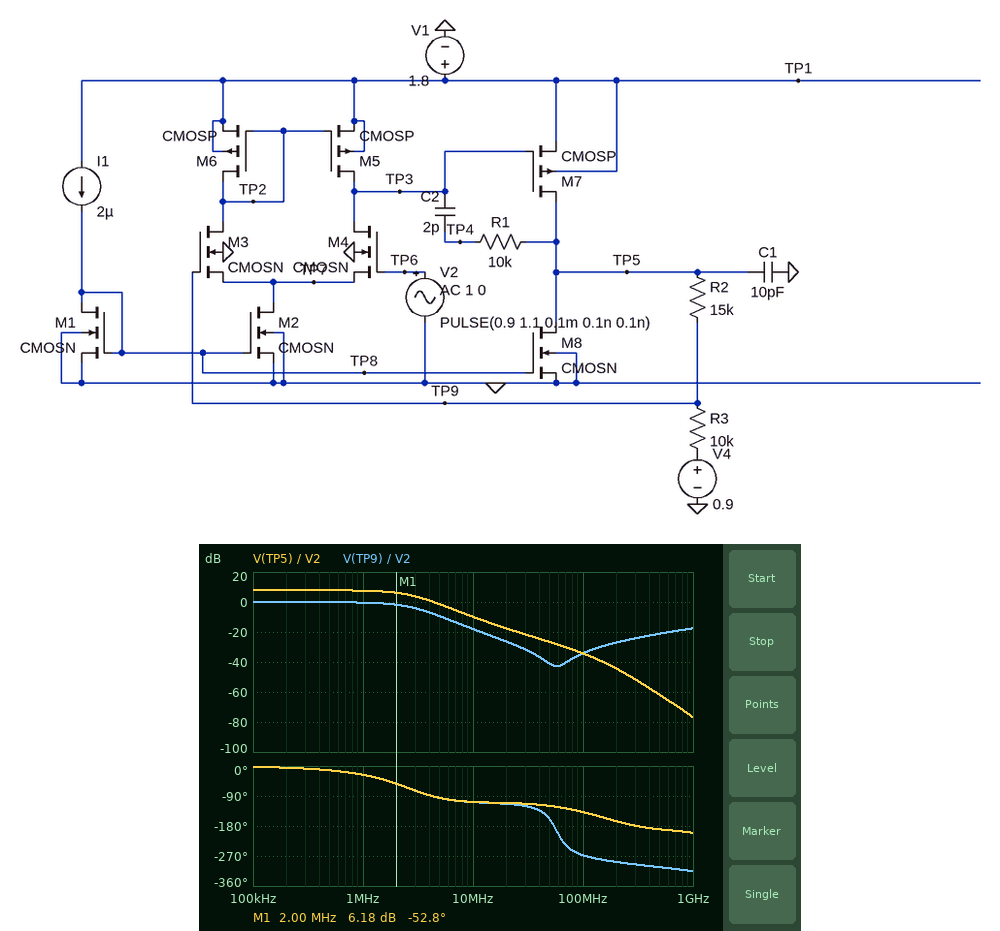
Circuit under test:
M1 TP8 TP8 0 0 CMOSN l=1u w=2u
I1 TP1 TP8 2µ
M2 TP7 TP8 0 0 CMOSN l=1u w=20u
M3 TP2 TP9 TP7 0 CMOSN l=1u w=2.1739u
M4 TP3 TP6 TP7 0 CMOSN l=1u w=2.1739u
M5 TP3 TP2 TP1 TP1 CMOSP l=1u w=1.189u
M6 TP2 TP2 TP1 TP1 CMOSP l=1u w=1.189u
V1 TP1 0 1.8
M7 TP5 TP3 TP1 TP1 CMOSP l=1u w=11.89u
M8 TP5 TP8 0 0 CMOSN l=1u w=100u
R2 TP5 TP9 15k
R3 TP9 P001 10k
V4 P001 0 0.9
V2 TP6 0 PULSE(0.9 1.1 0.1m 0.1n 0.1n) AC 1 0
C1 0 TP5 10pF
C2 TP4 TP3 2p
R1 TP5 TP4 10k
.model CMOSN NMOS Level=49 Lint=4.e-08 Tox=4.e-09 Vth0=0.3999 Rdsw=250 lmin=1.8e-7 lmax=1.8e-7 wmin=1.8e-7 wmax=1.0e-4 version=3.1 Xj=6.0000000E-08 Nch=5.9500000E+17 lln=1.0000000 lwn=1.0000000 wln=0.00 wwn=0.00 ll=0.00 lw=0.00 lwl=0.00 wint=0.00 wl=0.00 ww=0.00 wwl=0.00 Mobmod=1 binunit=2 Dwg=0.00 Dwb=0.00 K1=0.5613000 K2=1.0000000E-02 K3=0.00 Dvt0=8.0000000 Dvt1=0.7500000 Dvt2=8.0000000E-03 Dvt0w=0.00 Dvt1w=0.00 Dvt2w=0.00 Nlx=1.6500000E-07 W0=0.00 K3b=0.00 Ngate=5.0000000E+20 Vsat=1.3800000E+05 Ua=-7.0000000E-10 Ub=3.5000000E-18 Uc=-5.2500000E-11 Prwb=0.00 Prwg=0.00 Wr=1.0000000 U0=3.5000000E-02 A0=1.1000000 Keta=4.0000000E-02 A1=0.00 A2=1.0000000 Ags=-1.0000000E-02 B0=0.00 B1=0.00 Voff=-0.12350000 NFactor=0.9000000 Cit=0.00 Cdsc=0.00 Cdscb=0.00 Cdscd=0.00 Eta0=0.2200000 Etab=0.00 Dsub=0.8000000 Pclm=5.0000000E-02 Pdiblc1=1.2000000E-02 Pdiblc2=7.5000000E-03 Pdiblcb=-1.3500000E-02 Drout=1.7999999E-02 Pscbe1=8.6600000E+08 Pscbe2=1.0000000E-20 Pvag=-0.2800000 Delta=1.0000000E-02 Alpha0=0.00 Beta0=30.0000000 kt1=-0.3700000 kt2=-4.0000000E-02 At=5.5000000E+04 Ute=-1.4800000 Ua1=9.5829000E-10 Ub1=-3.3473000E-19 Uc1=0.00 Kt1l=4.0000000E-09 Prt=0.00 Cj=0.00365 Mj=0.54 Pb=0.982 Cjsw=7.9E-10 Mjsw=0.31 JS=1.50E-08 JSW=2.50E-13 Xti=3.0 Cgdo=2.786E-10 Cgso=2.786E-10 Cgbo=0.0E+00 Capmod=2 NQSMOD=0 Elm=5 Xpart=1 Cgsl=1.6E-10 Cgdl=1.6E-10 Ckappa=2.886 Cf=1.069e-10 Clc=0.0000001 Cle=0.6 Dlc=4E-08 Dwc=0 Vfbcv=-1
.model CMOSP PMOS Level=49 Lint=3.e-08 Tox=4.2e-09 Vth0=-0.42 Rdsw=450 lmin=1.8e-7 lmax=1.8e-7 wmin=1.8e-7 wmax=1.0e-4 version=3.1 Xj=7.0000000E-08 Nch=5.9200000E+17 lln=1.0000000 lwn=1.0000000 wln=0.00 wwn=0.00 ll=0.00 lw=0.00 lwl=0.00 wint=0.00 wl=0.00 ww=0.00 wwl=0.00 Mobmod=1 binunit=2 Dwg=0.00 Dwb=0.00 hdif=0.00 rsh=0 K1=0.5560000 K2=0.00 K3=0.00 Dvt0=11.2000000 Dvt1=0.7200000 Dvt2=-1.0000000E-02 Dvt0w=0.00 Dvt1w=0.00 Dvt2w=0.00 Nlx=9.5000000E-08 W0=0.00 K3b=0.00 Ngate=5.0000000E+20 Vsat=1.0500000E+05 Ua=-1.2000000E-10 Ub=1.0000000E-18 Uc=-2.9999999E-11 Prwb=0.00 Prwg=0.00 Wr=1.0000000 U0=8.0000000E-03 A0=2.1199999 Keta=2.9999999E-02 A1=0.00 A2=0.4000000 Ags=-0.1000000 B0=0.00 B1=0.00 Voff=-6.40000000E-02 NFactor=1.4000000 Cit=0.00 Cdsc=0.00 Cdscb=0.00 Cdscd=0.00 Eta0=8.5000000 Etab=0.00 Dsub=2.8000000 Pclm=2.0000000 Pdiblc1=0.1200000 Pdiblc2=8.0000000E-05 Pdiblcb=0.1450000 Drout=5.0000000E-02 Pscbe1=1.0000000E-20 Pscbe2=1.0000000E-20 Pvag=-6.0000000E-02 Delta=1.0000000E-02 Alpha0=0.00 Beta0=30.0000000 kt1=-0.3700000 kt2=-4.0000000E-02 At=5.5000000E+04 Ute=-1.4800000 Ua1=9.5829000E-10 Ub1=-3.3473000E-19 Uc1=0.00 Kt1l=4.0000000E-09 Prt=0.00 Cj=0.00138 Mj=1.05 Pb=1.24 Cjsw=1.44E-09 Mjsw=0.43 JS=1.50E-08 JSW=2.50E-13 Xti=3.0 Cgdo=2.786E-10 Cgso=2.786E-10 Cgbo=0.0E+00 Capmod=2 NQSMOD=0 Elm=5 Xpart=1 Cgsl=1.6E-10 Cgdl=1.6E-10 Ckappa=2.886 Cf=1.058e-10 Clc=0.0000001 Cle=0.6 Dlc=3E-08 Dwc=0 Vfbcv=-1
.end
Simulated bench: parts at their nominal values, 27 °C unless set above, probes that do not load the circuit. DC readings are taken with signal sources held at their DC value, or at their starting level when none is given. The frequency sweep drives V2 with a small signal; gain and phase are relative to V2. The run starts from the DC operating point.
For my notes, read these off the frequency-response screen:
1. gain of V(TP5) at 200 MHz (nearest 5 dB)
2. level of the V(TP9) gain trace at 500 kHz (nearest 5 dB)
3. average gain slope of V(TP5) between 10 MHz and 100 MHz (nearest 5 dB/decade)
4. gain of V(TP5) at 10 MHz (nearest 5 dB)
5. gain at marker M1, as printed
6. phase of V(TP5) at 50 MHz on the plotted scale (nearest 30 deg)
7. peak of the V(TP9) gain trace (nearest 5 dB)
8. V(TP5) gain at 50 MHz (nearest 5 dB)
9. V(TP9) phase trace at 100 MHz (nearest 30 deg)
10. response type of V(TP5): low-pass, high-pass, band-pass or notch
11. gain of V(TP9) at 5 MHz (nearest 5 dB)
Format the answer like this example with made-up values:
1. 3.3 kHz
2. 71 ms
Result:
1. -45 dB
2. 0 dB
3. -25 dB/decade
4. -10 dB
5. 6.18 dB
6. -120 deg
7. 0 dB
8. -25 dB
9. -270 deg
10. low-pass
11. -10 dB
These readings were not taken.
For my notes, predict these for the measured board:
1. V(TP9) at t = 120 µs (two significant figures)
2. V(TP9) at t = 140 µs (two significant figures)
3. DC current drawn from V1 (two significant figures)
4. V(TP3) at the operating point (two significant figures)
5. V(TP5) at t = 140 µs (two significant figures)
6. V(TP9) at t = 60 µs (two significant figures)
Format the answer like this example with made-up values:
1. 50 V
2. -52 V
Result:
1. 1.1 V
2. 1.1 V
3. 130 µA
4. 720 mV
5. 1.4 V
6. 900 mV
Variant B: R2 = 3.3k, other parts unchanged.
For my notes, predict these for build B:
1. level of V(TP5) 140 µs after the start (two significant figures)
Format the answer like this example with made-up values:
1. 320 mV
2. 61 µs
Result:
1. 1.2 V
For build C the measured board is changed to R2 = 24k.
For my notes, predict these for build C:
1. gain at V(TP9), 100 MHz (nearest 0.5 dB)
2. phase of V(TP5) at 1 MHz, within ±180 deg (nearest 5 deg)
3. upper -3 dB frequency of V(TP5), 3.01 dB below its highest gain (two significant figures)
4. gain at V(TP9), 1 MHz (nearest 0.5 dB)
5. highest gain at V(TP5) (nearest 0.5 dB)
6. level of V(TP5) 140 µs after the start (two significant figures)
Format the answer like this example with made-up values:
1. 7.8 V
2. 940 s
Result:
1. -32.0 dB
2. -35 deg
3. 2.0 MHz
4. -1.0 dB
5. 10.5 dB
6. 1.5 V
